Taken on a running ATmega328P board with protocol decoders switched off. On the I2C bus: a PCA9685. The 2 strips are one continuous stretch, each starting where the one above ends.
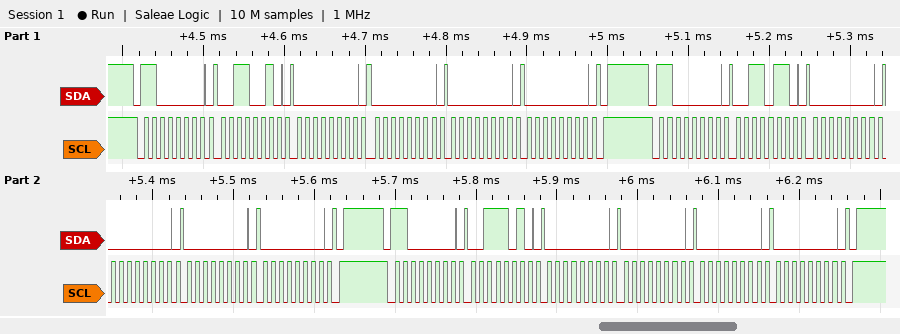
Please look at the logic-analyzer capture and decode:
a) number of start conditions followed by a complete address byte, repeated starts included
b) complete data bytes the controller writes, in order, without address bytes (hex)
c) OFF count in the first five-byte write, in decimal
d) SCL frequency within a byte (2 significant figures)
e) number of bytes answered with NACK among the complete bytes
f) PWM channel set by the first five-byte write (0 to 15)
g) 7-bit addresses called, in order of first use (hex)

3
32 00 00 00 00 36 00 00 00 00 3A 00 00 00 00
0
100 kHz
0
11
0x60
